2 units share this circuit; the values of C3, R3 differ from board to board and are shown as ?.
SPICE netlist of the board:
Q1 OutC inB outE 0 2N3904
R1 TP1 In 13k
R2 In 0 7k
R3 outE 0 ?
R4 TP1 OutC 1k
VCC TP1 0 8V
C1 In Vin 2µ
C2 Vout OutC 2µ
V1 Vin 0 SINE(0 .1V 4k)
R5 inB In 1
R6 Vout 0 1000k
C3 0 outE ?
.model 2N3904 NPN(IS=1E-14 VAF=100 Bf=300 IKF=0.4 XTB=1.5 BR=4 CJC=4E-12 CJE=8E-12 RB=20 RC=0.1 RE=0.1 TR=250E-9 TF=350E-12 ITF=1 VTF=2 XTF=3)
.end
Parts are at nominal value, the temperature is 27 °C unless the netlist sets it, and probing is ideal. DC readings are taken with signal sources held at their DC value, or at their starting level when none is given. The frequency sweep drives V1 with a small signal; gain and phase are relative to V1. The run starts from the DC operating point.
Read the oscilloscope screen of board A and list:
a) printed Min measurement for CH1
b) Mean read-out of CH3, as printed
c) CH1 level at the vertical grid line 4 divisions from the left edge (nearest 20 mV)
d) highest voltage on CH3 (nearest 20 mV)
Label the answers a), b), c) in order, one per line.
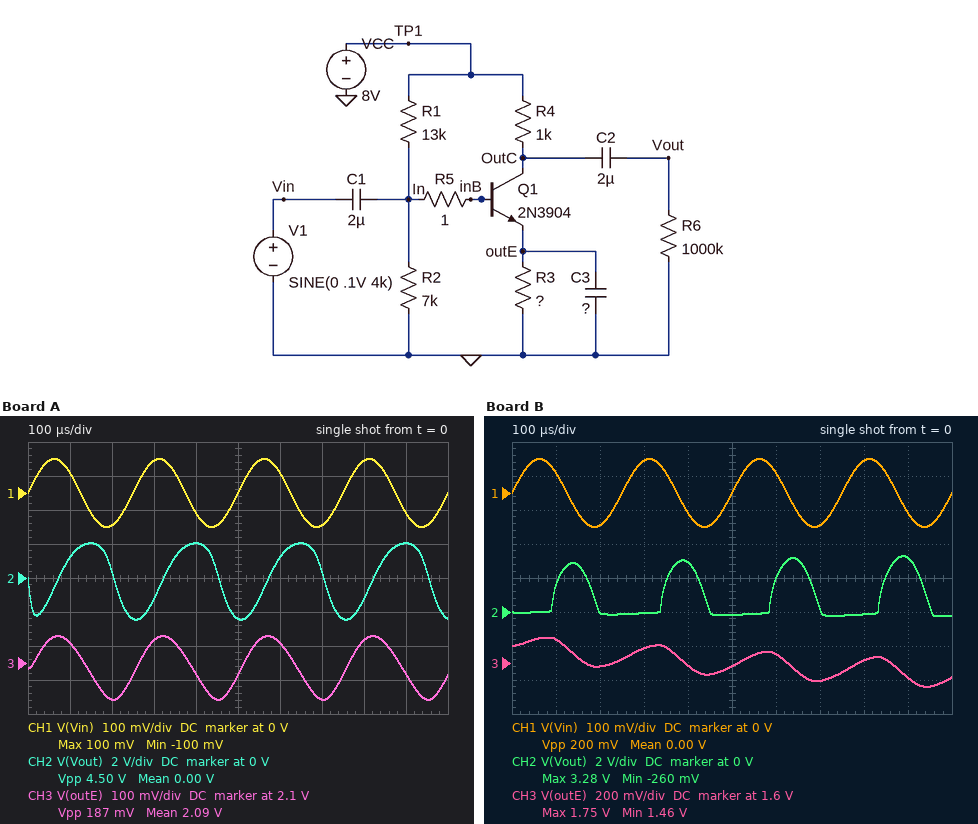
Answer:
a) -100 mV
b) 2.09 V
c) -60 mV
d) 2.18 V
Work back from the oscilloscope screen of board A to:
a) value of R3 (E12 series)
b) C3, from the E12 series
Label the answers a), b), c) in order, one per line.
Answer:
a) 820 Ω
b) 1 µF
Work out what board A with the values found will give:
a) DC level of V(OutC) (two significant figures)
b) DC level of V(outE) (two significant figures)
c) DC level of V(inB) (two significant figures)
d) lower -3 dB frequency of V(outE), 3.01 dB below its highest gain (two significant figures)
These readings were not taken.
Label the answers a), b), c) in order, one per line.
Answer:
a) 5.5 V
b) 2.1 V
c) 2.8 V
d) 18 Hz
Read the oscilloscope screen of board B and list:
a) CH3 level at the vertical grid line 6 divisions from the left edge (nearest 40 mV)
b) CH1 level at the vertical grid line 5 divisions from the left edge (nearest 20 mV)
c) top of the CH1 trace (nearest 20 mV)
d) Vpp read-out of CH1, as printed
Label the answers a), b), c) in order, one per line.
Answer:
a) 1.64 V
b) 0 V
c) 100 mV
d) 200 mV
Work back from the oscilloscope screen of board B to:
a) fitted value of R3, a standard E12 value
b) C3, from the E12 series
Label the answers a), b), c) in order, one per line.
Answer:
a) 270 Ω
b) 1.2 µF
